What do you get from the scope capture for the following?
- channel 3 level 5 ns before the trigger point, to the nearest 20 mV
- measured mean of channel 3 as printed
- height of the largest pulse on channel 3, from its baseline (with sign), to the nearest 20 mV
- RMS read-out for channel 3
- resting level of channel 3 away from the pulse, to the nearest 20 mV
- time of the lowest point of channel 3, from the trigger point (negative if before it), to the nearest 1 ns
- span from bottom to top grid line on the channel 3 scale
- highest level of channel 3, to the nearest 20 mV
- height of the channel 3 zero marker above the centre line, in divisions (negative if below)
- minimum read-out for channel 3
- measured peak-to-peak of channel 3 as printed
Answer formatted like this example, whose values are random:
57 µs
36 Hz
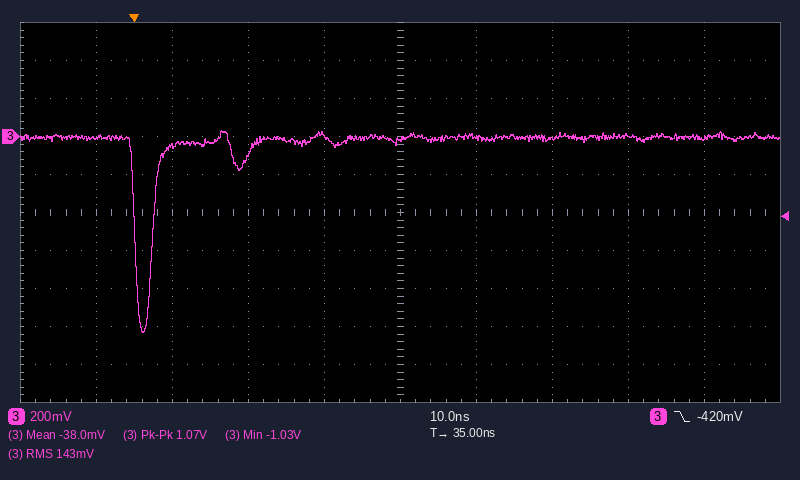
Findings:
0 mV
-38.0 mV
-1.02 V
143 mV
0 mV
+1 ns
2 V
40 mV
+2.0 div
-1.03 V
1.07 V
